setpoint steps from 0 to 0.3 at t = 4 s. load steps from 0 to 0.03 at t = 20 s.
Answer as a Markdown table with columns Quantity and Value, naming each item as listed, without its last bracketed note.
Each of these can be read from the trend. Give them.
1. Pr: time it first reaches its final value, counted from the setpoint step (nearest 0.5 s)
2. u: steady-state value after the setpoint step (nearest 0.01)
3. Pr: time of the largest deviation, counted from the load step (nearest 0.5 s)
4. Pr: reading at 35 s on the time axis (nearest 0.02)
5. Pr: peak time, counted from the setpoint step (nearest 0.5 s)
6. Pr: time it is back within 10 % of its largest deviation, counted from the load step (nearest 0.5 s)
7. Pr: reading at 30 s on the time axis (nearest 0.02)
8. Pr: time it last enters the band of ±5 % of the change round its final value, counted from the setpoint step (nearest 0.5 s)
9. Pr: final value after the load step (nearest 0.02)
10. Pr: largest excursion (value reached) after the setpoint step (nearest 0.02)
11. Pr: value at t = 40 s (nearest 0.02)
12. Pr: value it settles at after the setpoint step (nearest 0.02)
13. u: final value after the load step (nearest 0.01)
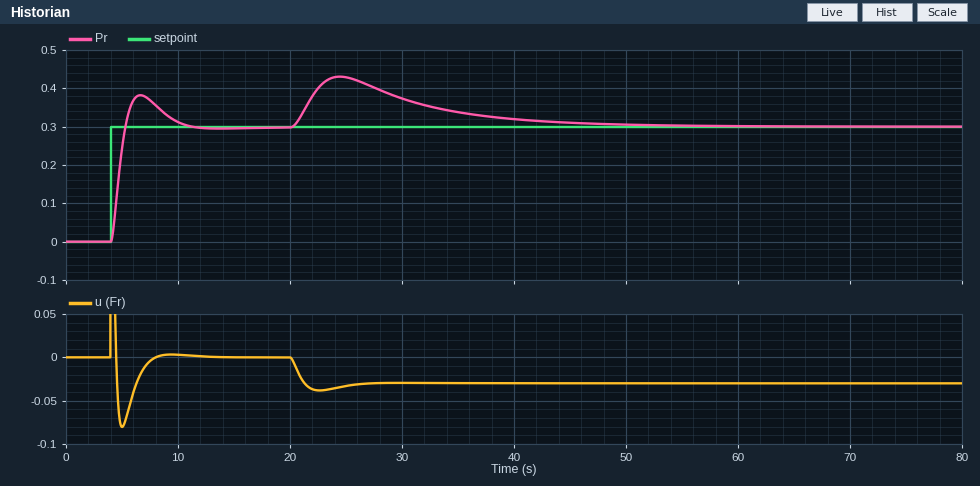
| Quantity | Value |
|---|---|
| Pr: time it first reaches its final value, counted from the setpoint step | 1.5 s |
| u: steady-state value after the setpoint step | 0.00 |
| Pr: time of the largest deviation, counted from the load step | 4.5 s |
| Pr: reading at 35 s on the time axis | 0.34 |
| Pr: peak time, counted from the setpoint step | 2.5 s |
| Pr: time it is back within 10 % of its largest deviation, counted from the load step | 23.0 s |
| Pr: reading at 30 s on the time axis | 0.38 |
| Pr: time it last enters the band of ±5 % of the change round its final value, counted from the setpoint step | 6.0 s |
| Pr: final value after the load step | 0.30 |
| Pr: largest excursion (value reached) after the setpoint step | 0.38 |
| Pr: value at t = 40 s | 0.32 |
| Pr: value it settles at after the setpoint step | 0.30 |
| u: final value after the load step | -0.03 |
